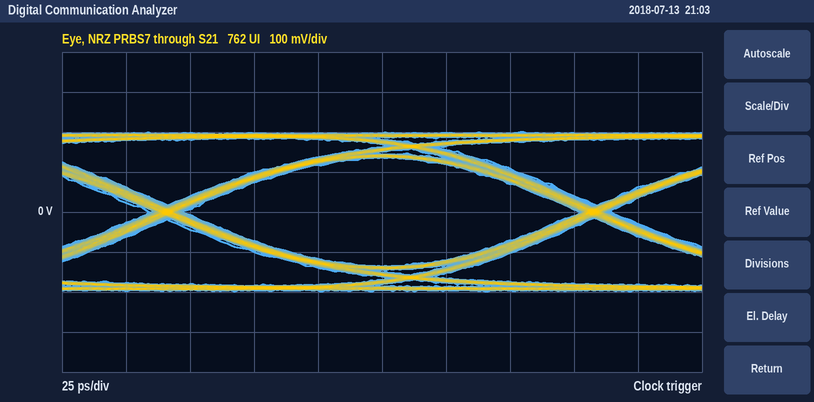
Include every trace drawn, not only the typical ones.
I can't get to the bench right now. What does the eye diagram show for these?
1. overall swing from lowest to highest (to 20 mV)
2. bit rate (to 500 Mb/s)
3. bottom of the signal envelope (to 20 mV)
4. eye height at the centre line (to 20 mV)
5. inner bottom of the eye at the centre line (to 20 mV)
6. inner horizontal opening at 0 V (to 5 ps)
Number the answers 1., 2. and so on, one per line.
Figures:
1. 400 mV
2. 6.0 Gb/s
3. -200 mV
4. 280 mV
5. -140 mV
6. 155 ps
